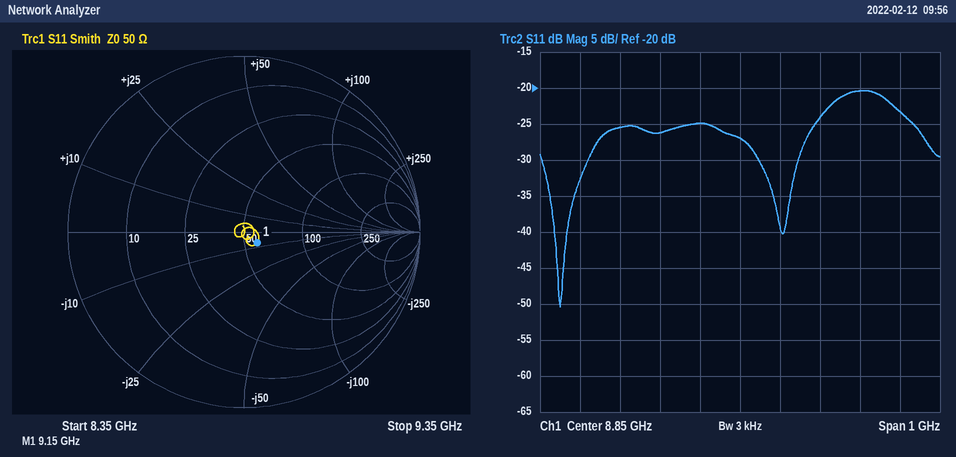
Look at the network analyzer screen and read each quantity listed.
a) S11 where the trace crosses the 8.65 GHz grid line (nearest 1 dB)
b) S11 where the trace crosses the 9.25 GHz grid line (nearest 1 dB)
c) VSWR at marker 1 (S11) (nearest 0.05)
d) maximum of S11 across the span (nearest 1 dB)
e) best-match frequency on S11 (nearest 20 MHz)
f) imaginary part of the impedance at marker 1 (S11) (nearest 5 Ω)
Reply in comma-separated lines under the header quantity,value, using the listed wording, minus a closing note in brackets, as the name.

quantity,value
S11 where the trace crosses the 8.65 GHz grid line,-26 dB
S11 where the trace crosses the 9.25 GHz grid line,-23 dB
VSWR at marker 1 (S11),1.20
maximum of S11 across the span,-20 dB
best-match frequency on S11,8.40 GHz
imaginary part of the impedance at marker 1 (S11),-5 Ω
